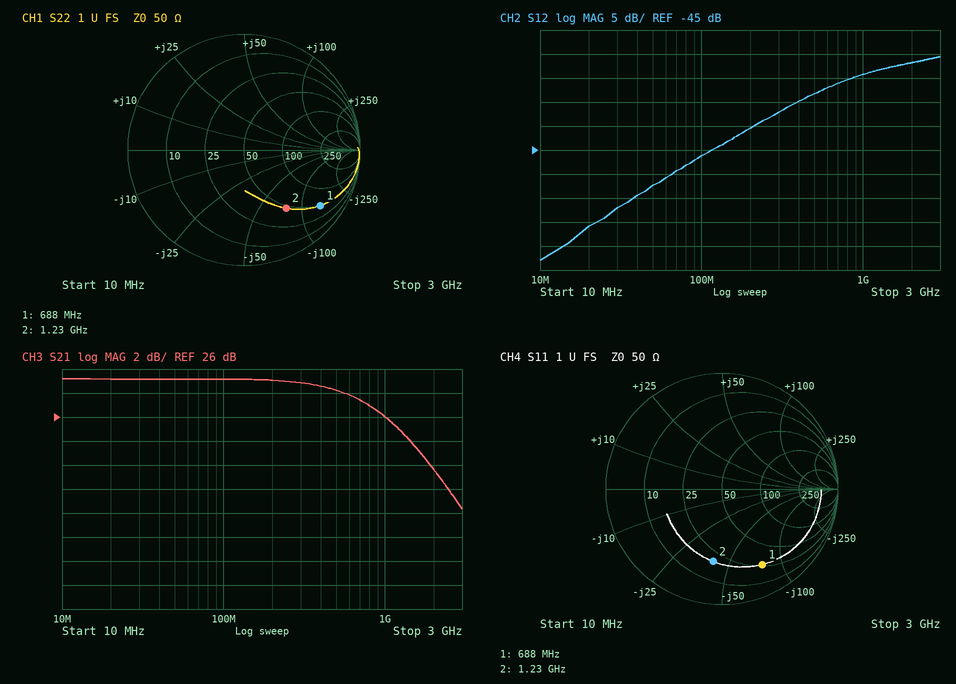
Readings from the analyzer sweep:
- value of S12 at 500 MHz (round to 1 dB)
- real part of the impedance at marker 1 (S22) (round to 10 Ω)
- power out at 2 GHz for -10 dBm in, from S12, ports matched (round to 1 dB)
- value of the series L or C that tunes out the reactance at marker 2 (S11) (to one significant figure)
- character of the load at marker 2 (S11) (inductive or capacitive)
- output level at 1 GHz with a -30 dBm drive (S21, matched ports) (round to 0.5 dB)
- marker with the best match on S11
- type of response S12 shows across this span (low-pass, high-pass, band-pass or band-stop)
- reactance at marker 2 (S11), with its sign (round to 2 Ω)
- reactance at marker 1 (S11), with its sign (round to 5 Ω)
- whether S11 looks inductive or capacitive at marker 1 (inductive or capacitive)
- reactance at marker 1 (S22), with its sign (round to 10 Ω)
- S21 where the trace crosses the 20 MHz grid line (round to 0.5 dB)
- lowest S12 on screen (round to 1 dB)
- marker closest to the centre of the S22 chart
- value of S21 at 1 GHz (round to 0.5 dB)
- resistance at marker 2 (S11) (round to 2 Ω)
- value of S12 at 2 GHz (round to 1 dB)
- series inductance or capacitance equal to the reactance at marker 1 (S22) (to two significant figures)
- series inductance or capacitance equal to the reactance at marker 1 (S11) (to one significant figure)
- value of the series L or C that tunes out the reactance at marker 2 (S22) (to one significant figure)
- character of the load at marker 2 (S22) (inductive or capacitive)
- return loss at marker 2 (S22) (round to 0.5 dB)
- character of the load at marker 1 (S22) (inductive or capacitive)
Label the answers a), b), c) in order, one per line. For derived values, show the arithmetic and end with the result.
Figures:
a) -33 dB
b) 50 Ω
c) -10 dBm + (-27 dB) = -37 dBm
d) L = 40 Ω/(2π × 1.23 GHz) ≈ 5 nH
e) capacitive
f) -30 dBm + (26.0 dB) = -4.0 dBm
g) marker 2
h) high-pass
i) -40 Ω
j) -75 Ω
k) capacitive
l) -140 Ω
m) 29.0 dB
n) -68 dB
o) marker 2
p) 26.0 dB
q) 20 Ω
r) -27 dB
s) C = 1/(2π × 688 MHz × 140 Ω) ≈ 1.7 pF
t) C = 1/(2π × 688 MHz × 75 Ω) ≈ 3 pF
u) L = 75 Ω/(2π × 1.23 GHz) ≈ 10 nH
v) capacitive
w) 4.0 dB
x) capacitive
